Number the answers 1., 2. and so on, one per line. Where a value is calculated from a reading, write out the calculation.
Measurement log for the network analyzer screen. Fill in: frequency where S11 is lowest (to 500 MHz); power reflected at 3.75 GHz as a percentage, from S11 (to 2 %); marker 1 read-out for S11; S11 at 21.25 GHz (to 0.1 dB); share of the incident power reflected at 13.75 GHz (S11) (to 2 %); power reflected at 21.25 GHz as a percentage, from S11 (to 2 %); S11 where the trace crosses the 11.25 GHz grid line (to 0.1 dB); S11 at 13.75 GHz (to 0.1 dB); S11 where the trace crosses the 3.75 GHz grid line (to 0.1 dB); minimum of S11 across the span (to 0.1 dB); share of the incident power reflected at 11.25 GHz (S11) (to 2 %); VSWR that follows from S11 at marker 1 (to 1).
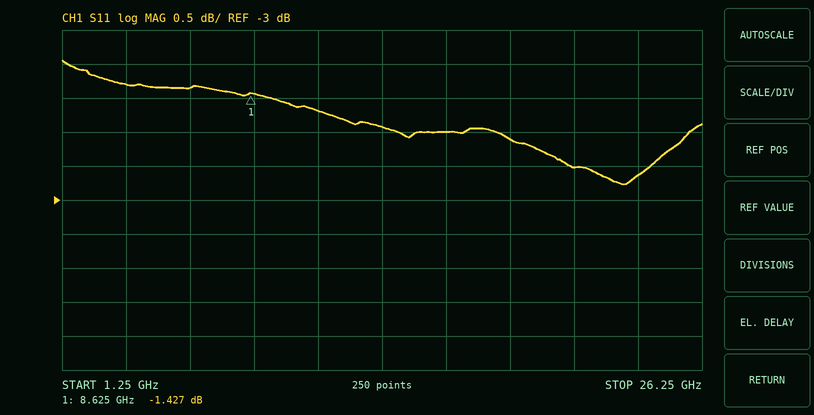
1. 23.0 GHz
2. 10^(-1.3/10) ≈ 74 %
3. -1.427 dB
4. -2.5 dB
5. 10^(-1.9/10) ≈ 64.6 %, so 64 % to the nearest 2 %
6. 10^(-2.5/10) ≈ 56 %
7. -1.7 dB
8. -1.9 dB
9. -1.3 dB
10. -2.8 dB
11. 10^(-1.7/10) ≈ 68 %
12. (1 + 0.8485)/(1 − 0.8485) ≈ 12
